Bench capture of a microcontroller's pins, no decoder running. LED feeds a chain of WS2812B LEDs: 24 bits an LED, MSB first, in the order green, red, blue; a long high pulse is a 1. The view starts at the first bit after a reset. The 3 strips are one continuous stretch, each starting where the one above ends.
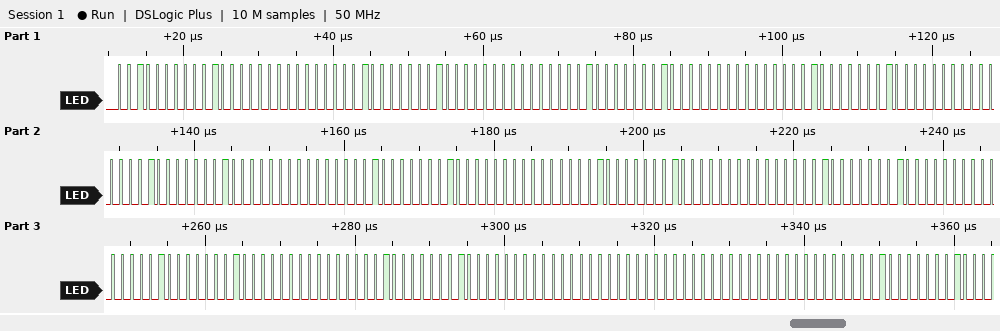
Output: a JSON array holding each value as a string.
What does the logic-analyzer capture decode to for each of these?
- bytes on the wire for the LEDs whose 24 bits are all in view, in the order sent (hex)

["20 20 00 20 20 00 20 20 00 20 20 00 20 20 00 20 20 00 20 20 00 20 20 00 20 20 00 20 20 00 00 00 00"]
